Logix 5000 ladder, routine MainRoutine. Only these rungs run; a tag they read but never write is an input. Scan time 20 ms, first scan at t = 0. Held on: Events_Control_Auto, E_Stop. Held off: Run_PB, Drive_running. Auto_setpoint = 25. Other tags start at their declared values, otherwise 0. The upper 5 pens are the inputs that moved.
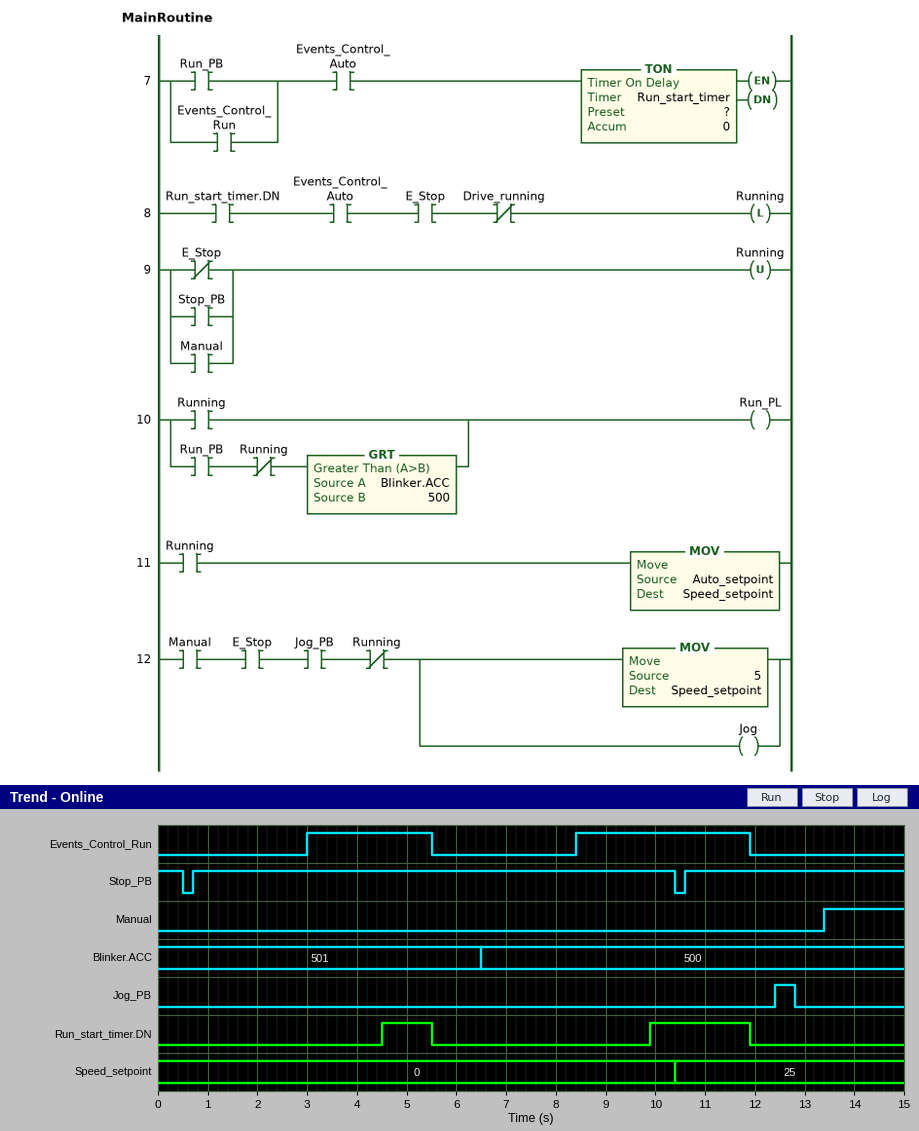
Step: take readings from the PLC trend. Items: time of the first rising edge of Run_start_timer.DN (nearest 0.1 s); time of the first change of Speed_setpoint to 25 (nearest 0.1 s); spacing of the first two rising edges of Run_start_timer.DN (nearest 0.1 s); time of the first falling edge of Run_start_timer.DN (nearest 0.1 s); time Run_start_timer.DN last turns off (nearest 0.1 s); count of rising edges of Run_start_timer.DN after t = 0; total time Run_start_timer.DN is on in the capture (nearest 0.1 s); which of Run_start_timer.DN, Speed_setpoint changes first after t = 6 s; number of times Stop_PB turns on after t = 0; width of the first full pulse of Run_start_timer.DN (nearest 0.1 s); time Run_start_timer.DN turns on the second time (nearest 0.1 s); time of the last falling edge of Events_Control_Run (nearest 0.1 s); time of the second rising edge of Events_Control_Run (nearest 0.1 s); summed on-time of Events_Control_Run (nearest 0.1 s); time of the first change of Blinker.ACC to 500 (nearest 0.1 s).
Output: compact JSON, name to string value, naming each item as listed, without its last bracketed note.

{"time of the first rising edge of Run_start_timer.DN": "4.5 s", "time of the first change of Speed_setpoint to 25": "10.4 s", "spacing of the first two rising edges of Run_start_timer.DN": "5.4 s", "time of the first falling edge of Run_start_timer.DN": "5.5 s", "time Run_start_timer.DN last turns off": "11.9 s", "count of rising edges of Run_start_timer.DN after t = 0": "2", "total time Run_start_timer.DN is on in the capture": "3.0 s", "which of Run_start_timer.DN, Speed_setpoint changes first after t = 6 s": "Run_start_timer.DN", "number of times Stop_PB turns on after t = 0": "2", "width of the first full pulse of Run_start_timer.DN": "1.0 s", "time Run_start_timer.DN turns on the second time": "9.9 s", "time of the last falling edge of Events_Control_Run": "11.9 s", "time of the second rising edge of Events_Control_Run": "8.4 s", "summed on-time of Events_Control_Run": "6.0 s", "time of the first change of Blinker.ACC to 500": "6.5 s"}
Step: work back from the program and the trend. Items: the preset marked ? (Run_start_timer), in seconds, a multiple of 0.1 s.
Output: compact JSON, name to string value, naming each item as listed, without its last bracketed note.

{"the preset marked ? (Run_start_timer), in seconds, a multiple of 0.1 s": "1.5 s"}
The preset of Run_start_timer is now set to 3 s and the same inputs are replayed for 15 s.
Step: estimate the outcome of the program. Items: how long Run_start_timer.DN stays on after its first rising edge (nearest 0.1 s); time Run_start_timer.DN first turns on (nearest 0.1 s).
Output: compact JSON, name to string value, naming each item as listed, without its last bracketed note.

{"how long Run_start_timer.DN stays on after its first rising edge": "0.5 s", "time Run_start_timer.DN first turns on": "11.4 s"}
